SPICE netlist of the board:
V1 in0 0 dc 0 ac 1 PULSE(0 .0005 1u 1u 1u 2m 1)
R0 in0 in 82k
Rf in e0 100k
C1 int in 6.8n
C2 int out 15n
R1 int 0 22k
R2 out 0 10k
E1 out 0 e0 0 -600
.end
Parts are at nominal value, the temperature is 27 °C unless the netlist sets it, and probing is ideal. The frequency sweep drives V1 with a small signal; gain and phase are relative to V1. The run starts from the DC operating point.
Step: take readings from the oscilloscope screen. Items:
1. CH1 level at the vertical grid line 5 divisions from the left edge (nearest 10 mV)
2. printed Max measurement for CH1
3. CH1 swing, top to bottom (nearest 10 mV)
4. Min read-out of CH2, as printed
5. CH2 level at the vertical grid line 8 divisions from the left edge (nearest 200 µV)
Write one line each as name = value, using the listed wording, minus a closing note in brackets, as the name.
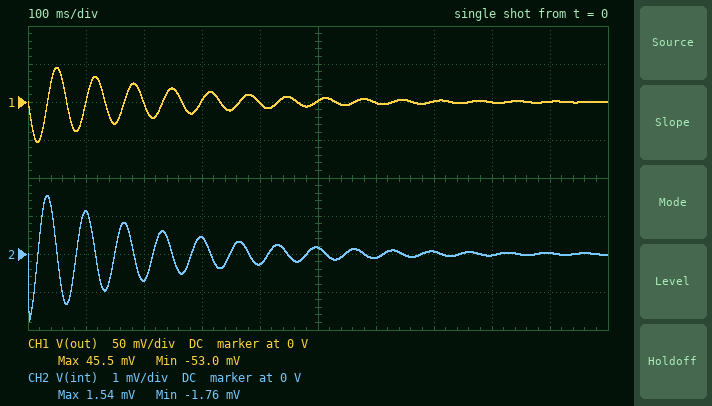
CH1 level at the vertical grid line 5 divisions from the left edge = 0 V
printed Max measurement for CH1 = 45.5 mV
CH1 swing, top to bottom = 100 mV
Min read-out of CH2, as printed = -1.76 mV
CH2 level at the vertical grid line 8 divisions from the left edge = 0 V
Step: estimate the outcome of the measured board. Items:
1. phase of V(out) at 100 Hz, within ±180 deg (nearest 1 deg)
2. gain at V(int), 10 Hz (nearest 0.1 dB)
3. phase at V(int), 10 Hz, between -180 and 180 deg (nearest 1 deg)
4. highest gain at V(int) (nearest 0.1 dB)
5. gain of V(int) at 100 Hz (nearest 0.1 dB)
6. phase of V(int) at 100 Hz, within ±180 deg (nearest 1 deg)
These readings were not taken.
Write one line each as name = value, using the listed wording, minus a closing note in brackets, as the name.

phase of V(out) at 100 Hz, within ±180 deg = 18 deg
gain at V(int), 10 Hz = 26.8 dB
phase at V(int), 10 Hz, between -180 and 180 deg = -97 deg
highest gain at V(int) = 45.6 dB
gain of V(int) at 100 Hz = 9.3 dB
phase of V(int) at 100 Hz, within ±180 deg = 91 deg
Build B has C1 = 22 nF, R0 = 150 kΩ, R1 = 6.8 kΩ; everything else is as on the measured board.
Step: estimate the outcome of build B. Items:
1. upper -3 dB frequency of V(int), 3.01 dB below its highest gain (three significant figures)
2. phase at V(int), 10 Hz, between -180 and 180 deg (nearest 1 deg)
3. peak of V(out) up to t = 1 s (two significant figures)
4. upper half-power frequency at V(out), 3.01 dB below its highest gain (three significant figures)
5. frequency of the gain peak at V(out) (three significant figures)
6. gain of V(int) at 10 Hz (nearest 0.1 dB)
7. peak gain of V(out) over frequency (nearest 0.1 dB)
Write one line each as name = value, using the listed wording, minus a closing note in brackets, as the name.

upper -3 dB frequency of V(int), 3.01 dB below its highest gain = 12.7 Hz
phase at V(int), 10 Hz, between -180 and 180 deg = -138 deg
peak of V(out) up to t = 1 s = 24 mV
upper half-power frequency at V(out), 3.01 dB below its highest gain = 12.3 Hz
frequency of the gain peak at V(out) = 11.0 Hz
gain of V(int) at 10 Hz = 22.1 dB
peak gain of V(out) over frequency = 67.7 dB
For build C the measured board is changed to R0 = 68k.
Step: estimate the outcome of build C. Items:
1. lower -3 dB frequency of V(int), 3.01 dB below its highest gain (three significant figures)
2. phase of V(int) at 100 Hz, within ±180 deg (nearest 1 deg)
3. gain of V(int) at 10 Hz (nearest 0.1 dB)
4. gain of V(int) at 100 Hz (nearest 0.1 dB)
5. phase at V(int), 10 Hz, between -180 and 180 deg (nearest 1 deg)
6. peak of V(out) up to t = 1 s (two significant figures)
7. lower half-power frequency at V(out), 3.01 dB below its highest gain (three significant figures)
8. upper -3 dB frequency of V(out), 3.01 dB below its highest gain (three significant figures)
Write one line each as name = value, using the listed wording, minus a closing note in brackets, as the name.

lower -3 dB frequency of V(int), 3.01 dB below its highest gain = 15.8 Hz
phase of V(int) at 100 Hz, within ±180 deg = 91 deg
gain of V(int) at 10 Hz = 25.8 dB
gain of V(int) at 100 Hz = 11.0 dB
phase at V(int), 10 Hz, between -180 and 180 deg = -95 deg
peak of V(out) up to t = 1 s = 50 mV
lower half-power frequency at V(out), 3.01 dB below its highest gain = 15.7 Hz
upper -3 dB frequency of V(out), 3.01 dB below its highest gain = 17.4 Hz
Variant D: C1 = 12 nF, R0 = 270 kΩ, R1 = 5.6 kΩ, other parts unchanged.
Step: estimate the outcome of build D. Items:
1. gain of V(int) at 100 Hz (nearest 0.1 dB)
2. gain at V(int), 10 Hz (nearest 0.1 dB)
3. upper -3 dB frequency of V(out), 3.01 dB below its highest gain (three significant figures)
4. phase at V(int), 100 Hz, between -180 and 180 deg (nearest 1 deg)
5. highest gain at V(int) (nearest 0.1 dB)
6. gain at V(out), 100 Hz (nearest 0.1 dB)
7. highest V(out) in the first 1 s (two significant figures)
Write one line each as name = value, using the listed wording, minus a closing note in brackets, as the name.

gain of V(int) at 100 Hz = -6.1 dB
gain at V(int), 10 Hz = 17.7 dB
upper -3 dB frequency of V(out), 3.01 dB below its highest gain = 13.8 Hz
phase at V(int), 100 Hz, between -180 and 180 deg = 92 deg
highest gain at V(int) = 23.4 dB
gain at V(out), 100 Hz = 19.5 dB
highest V(out) in the first 1 s = 25 mV
